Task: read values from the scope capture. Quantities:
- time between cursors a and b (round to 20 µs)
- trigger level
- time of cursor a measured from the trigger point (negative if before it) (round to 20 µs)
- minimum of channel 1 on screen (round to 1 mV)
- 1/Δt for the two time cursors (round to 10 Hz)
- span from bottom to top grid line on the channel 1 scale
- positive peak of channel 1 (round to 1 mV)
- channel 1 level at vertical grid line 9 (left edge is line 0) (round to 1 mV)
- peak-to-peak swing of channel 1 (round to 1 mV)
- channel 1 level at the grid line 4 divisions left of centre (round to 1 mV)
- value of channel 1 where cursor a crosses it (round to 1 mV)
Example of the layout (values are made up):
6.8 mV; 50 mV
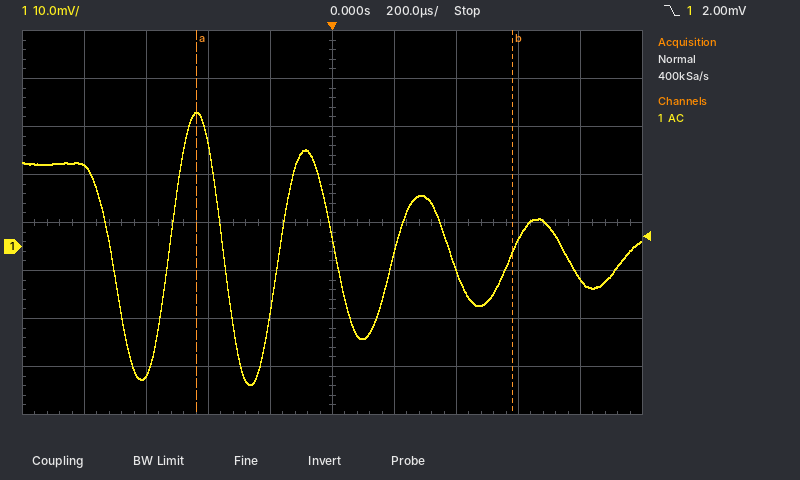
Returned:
1.02 ms; 2.00 mV; -440 µs; -29 mV; 980 Hz; 80 mV; 28 mV; -7 mV; 57 mV; 17 mV; 28 mV
